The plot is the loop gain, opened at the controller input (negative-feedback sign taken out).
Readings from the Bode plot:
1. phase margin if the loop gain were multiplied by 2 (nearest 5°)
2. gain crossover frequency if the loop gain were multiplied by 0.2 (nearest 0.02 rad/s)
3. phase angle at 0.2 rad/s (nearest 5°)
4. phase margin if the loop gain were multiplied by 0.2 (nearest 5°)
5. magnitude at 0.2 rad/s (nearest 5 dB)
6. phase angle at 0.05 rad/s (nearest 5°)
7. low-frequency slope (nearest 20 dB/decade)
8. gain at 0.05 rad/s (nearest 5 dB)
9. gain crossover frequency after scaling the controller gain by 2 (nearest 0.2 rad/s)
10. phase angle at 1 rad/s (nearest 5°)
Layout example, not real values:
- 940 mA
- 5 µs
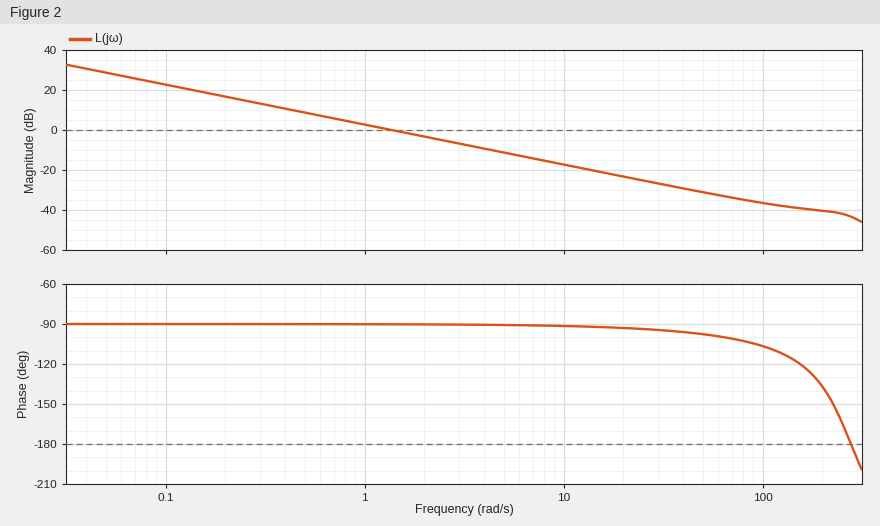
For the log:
- 90°
- 0.28 rad/s
- -90°
- 90°
- 15 dB
- -90°
- -20 dB/decade
- 30 dB
- 2.8 rad/s
- -90°
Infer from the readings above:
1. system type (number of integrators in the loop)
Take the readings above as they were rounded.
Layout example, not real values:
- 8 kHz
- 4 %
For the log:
- 1
